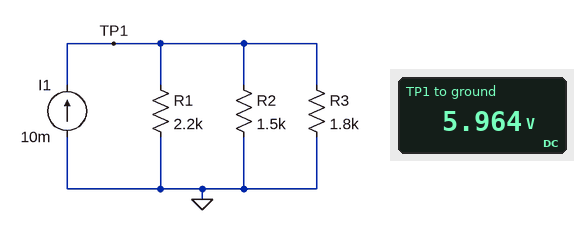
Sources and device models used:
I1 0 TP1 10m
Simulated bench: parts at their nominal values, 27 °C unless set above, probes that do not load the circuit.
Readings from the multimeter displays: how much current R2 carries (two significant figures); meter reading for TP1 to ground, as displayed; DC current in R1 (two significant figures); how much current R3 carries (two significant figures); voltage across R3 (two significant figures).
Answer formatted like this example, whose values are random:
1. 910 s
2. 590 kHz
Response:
1. 4.0 mA
2. 5.964 V
3. 2.7 mA
4. 3.3 mA
5. 6.0 V
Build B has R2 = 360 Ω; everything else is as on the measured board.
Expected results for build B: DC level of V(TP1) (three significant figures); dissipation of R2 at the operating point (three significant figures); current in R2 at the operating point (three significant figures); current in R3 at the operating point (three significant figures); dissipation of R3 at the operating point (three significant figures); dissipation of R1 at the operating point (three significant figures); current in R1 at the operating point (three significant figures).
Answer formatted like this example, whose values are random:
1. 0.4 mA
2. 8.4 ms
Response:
1. 2.64 V
2. 19.4 mW
3. 7.33 mA
4. 1.47 mA
5. 3.87 mW
6. 3.17 mW
7. 1.20 mA
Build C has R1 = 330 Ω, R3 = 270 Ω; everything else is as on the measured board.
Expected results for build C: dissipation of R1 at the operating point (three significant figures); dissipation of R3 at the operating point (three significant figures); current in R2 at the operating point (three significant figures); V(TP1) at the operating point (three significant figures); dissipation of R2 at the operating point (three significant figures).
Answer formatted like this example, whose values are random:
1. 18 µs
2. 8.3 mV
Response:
1. 5.53 mW
2. 6.76 mW
3. 901 µA
4. 1.35 V
5. 1.22 mW
